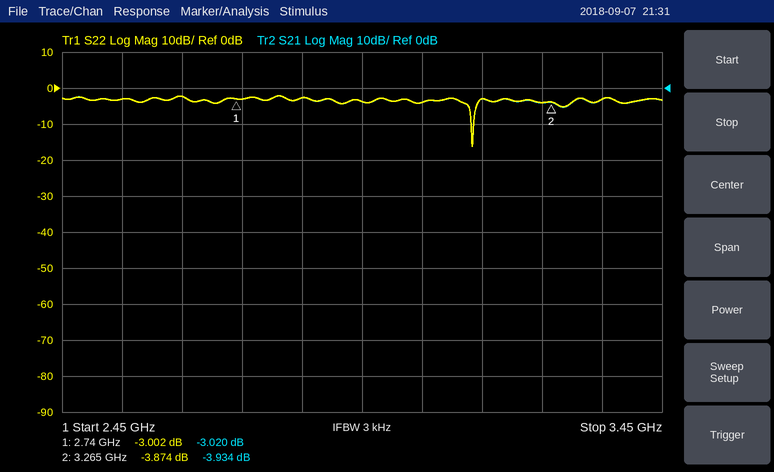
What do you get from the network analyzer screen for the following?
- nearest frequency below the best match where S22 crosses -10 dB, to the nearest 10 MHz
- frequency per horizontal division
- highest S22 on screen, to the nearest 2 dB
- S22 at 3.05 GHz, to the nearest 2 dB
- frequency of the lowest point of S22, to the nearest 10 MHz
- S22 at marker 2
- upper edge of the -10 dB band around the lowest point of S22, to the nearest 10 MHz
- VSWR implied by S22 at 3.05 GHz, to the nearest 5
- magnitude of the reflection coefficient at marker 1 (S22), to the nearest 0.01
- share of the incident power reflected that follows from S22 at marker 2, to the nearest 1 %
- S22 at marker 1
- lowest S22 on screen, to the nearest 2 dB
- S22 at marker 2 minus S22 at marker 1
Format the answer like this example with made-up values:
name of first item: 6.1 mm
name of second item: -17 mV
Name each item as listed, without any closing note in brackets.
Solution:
nearest frequency below the best match where S22 crosses -10 dB, to the nearest 10 MHz: 3.13 GHz
frequency per horizontal division: 100 MHz
highest S22 on screen, to the nearest 2 dB: -2 dB
S22 at 3.05 GHz, to the nearest 2 dB: -4 dB
frequency of the lowest point of S22, to the nearest 10 MHz: 3.13 GHz
S22 at marker 2: -3.874 dB
upper edge of the -10 dB band around the lowest point of S22, to the nearest 10 MHz: 3.14 GHz
VSWR implied by S22 at 3.05 GHz, to the nearest 5: 5
magnitude of the reflection coefficient at marker 1 (S22), to the nearest 0.01: 0.71
share of the incident power reflected that follows from S22 at marker 2, to the nearest 1 %: 41 %
S22 at marker 1: -3.002 dB
lowest S22 on screen, to the nearest 2 dB: -16 dB
S22 at marker 2 minus S22 at marker 1: -0.872 dB
